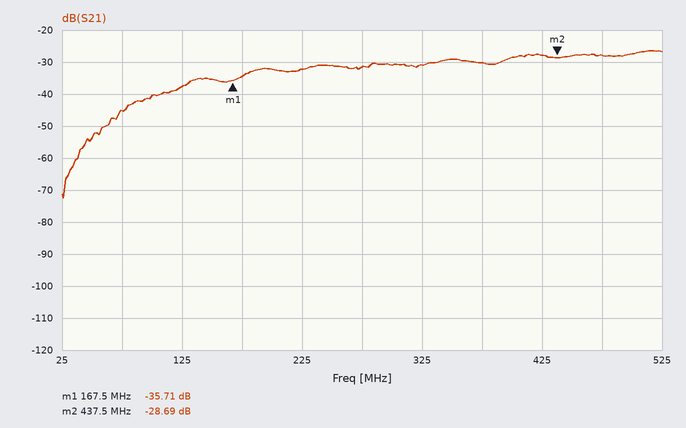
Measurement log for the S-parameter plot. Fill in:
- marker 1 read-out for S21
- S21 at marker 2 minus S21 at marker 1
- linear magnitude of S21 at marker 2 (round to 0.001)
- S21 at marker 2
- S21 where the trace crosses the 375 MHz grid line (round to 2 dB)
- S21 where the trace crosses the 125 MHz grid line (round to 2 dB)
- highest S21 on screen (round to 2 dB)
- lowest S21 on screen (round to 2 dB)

-35.71 dB
7.02 dB
0.037
-28.69 dB
-30 dB
-38 dB
-26 dB
-72 dB
